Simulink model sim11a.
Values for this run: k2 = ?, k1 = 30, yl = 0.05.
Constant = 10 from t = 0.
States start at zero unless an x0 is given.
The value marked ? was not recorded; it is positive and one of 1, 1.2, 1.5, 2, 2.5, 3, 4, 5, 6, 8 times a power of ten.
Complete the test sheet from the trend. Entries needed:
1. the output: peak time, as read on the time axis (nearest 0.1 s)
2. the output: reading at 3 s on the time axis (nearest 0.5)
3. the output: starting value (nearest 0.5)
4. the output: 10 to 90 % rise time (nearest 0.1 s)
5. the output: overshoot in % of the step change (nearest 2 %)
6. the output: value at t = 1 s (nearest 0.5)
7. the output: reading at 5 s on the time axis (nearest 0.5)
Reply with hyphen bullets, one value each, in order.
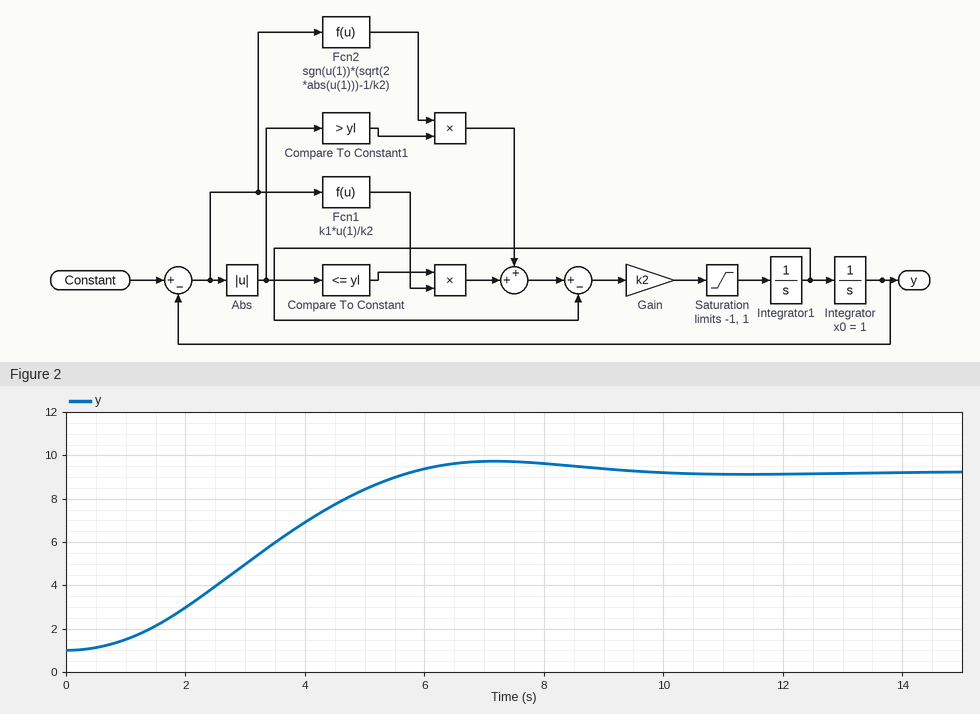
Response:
- 7.2 s
- 5.0
- 1.0
- 3.7 s
- 6 %
- 1.5
- 8.5
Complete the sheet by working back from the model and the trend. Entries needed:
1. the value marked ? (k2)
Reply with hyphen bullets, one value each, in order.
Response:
- 0.8
